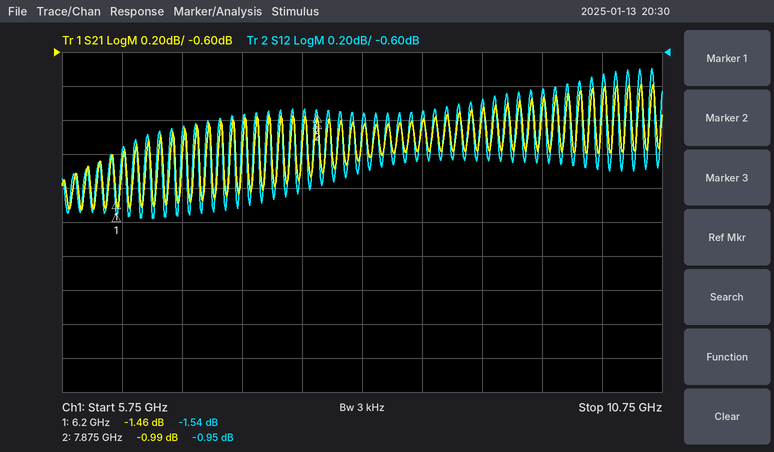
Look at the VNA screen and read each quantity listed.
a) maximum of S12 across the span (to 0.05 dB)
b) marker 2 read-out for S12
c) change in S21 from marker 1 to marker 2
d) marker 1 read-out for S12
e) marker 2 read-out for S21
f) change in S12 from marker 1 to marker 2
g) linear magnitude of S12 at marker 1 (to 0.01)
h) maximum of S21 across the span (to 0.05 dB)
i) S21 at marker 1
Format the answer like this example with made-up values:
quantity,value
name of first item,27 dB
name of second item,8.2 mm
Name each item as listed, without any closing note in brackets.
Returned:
quantity,value
maximum of S12 across the span,-0.70 dB
marker 2 read-out for S12,-0.95 dB
change in S21 from marker 1 to marker 2,0.47 dB
marker 1 read-out for S12,-1.54 dB
marker 2 read-out for S21,-0.99 dB
change in S12 from marker 1 to marker 2,0.59 dB
linear magnitude of S12 at marker 1,0.84
maximum of S21 across the span,-0.80 dB
S21 at marker 1,-1.46 dB
